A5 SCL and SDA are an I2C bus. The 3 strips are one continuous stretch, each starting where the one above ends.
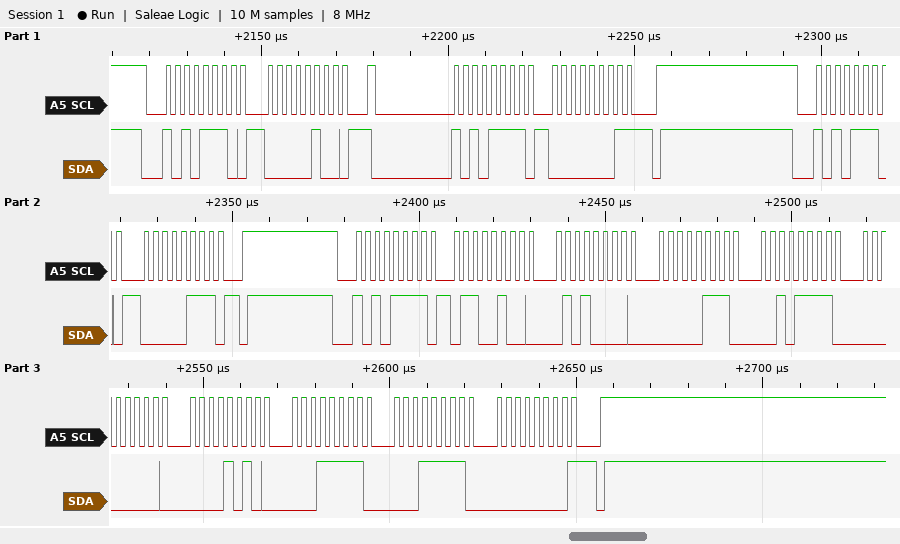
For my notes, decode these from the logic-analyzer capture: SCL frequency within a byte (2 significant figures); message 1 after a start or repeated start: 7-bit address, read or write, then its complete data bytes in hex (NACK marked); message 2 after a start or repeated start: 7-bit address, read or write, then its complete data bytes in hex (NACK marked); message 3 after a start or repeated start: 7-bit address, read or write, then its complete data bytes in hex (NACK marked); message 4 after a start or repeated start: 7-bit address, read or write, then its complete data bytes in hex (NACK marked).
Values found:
400 kHz
0x57 write: 04
0x57 read: 01 NACK
0x57 write: 07
0x57 read: 64 50 07 2F 00 0A 1F 1F 00 NACK
